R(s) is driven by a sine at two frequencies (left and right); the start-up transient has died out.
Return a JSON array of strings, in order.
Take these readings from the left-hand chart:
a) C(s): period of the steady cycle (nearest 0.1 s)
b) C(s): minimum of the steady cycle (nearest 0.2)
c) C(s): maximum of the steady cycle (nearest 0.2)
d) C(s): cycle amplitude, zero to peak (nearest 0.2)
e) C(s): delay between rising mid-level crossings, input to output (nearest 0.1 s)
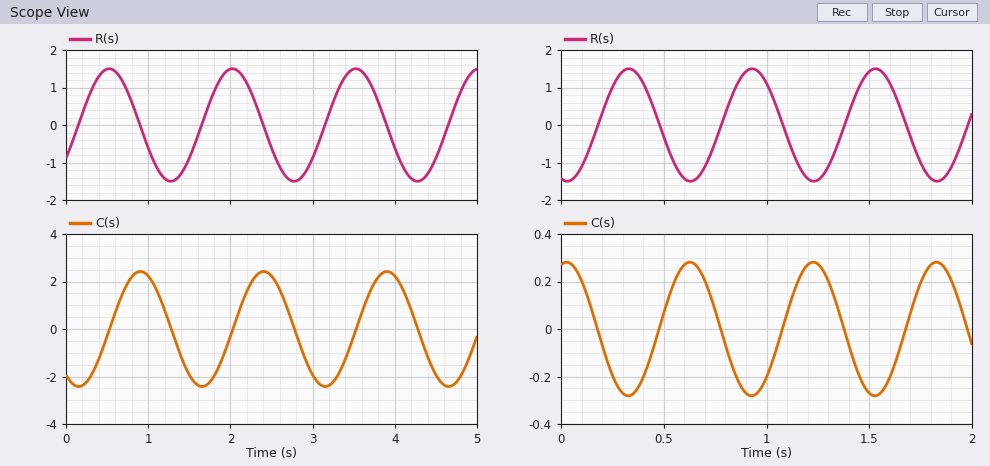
["1.5 s", "-2.4", "2.4", "2.4", "0.4 s"]
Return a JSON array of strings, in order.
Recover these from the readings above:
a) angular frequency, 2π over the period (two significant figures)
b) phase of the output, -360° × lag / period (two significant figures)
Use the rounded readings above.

["4.2 rad/s", "-96°"]
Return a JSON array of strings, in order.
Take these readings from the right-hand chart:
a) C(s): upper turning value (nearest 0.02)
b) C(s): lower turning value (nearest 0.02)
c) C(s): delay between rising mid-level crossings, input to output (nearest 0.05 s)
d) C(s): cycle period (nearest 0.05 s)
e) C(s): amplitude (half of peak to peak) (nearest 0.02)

["0.28", "-0.28", "0.30 s", "0.60 s", "0.28"]
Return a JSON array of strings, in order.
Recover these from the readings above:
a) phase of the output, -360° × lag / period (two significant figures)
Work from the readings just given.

["-180°"]
